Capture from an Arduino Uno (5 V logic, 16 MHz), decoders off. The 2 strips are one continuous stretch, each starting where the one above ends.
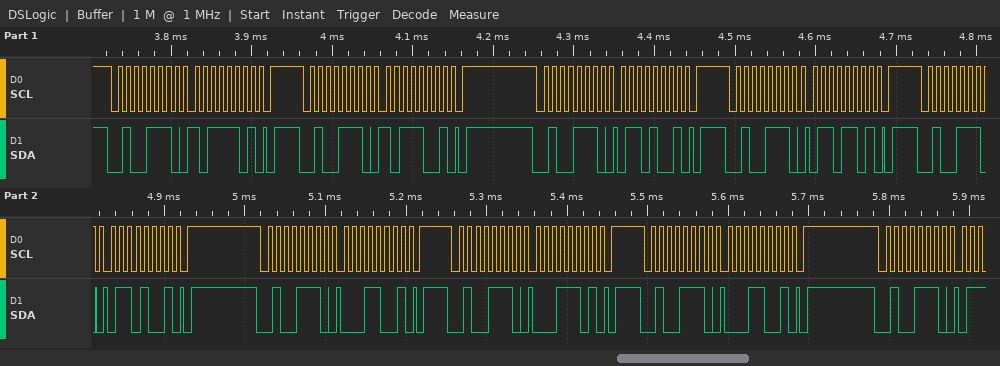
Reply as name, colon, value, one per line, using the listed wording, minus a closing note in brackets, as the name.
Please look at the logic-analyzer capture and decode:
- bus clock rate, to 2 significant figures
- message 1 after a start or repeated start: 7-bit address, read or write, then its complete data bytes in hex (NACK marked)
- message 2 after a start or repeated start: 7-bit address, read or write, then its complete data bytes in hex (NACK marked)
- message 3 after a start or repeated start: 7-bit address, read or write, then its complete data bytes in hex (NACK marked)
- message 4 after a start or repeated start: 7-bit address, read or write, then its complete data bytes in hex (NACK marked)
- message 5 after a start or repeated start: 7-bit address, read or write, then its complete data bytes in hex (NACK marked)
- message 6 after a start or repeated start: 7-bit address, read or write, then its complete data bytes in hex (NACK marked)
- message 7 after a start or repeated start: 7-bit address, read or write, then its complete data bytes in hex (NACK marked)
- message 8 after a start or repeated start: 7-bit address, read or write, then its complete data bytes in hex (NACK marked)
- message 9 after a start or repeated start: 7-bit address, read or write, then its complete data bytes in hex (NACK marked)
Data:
bus clock rate, to 2 significant figures: 100 kHz
message 1 after a start or repeated start: 7-bit address, read or write, then its complete data bytes in hex: 0x27 write: BD
message 2 after a start or repeated start: 7-bit address, read or write, then its complete data bytes in hex: 0x27 write: B9
message 3 after a start or repeated start: 7-bit address, read or write, then its complete data bytes in hex: 0x27 write: 69
message 4 after a start or repeated start: 7-bit address, read or write, then its complete data bytes in hex: 0x27 write: 6D
message 5 after a start or repeated start: 7-bit address, read or write, then its complete data bytes in hex: 0x27 write: 69
message 6 after a start or repeated start: 7-bit address, read or write, then its complete data bytes in hex: 0x27 write: 19
message 7 after a start or repeated start: 7-bit address, read or write, then its complete data bytes in hex: 0x27 write: 1D
message 8 after a start or repeated start: 7-bit address, read or write, then its complete data bytes in hex: 0x27 write: 19
message 9 after a start or repeated start: 7-bit address, read or write, then its complete data bytes in hex: 0x27 write
